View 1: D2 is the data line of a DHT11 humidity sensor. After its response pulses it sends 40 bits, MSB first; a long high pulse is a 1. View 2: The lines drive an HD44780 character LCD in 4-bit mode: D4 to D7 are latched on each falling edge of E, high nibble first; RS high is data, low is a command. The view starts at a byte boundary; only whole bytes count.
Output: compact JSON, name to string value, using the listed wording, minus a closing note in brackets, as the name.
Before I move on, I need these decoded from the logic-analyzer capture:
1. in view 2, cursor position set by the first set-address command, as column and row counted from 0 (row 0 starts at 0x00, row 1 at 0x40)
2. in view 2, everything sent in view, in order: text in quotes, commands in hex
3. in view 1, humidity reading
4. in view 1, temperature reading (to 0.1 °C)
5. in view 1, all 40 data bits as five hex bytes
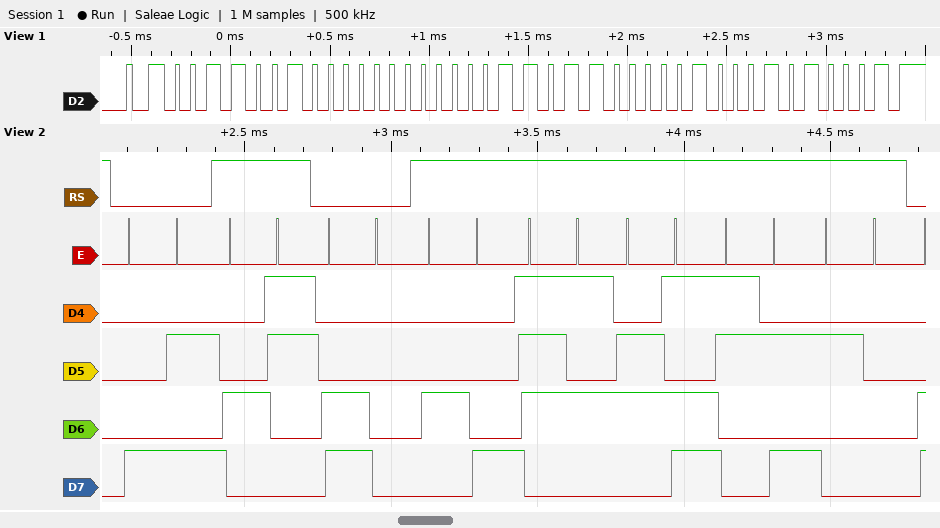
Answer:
{"in view 2, cursor position set by the first set-address command, as column and row counted from 0": "column 10, row 0", "in view 2, everything sent in view, in order: text in quotes, commands in hex": "0x8A \"C\" 0xC0 \"Hum: \"", "in view 1, humidity reading": "50 %", "in view 1, temperature reading": "27.4 °C", "in view 1, all 40 data bits as five hex bytes": "32 00 1B 04 51"}
